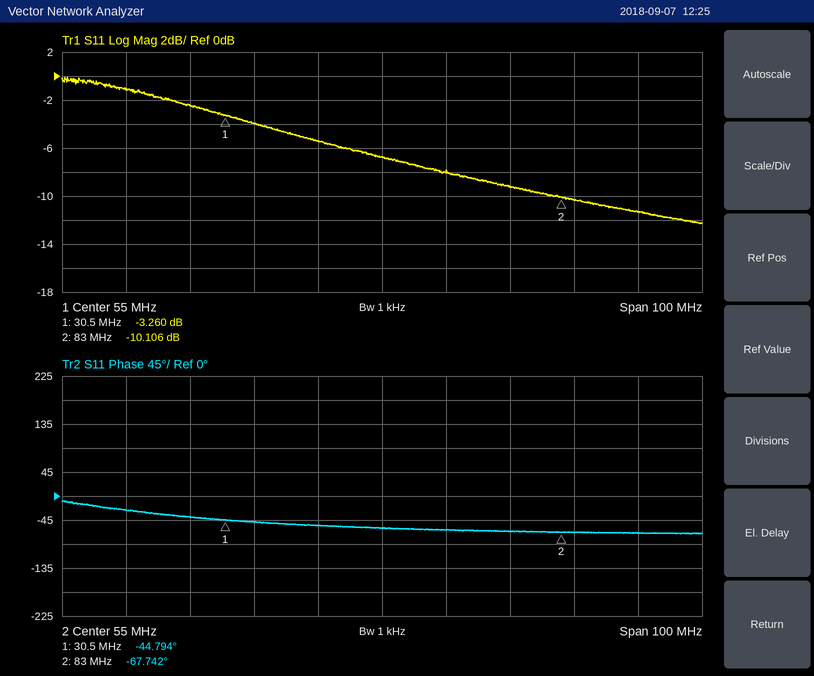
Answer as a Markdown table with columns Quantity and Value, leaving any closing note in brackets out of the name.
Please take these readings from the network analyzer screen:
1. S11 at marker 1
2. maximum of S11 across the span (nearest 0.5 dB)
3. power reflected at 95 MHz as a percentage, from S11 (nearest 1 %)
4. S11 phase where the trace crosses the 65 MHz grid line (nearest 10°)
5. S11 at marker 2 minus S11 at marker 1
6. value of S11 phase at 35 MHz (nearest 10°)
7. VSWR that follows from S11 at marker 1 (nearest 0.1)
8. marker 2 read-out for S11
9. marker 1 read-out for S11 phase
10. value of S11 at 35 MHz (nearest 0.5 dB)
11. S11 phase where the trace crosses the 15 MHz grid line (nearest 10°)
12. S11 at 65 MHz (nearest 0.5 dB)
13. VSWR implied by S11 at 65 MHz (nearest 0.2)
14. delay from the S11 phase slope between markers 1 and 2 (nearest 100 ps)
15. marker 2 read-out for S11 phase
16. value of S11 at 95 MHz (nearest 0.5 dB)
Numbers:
| Quantity | Value |
|---|---|
| S11 at marker 1 | -3.260 dB |
| maximum of S11 across the span | 0.0 dB |
| power reflected at 95 MHz as a percentage, from S11 | 7 % |
| S11 phase where the trace crosses the 65 MHz grid line | -60° |
| S11 at marker 2 minus S11 at marker 1 | -6.846 dB |
| value of S11 phase at 35 MHz | -50° |
| VSWR that follows from S11 at marker 1 | 5.4 |
| marker 2 read-out for S11 | -10.106 dB |
| marker 1 read-out for S11 phase | -44.794° |
| value of S11 at 35 MHz | -4.0 dB |
| S11 phase where the trace crosses the 15 MHz grid line | -30° |
| S11 at 65 MHz | -8.0 dB |
| VSWR implied by S11 at 65 MHz | 2.4 |
| delay from the S11 phase slope between markers 1 and 2 | 1.2 ns |
| marker 2 read-out for S11 phase | -67.742° |
| value of S11 at 95 MHz | -11.5 dB |
